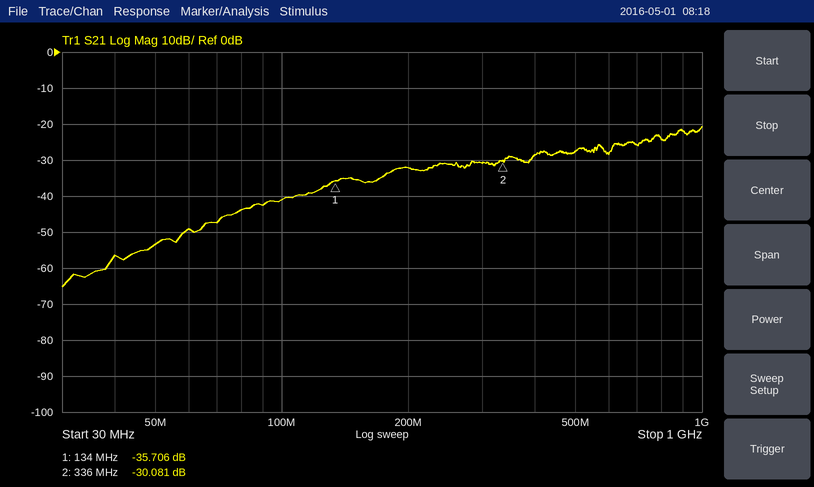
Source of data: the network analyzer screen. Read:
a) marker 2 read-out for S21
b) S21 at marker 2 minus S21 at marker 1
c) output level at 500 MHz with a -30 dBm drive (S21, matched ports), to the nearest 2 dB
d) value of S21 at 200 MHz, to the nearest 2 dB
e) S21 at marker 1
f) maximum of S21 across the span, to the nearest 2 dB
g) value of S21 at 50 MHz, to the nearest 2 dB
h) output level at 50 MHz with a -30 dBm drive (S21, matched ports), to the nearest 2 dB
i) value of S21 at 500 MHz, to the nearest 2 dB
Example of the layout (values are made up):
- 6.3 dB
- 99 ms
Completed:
- -30.081 dB
- 5.625 dB
- -58 dBm
- -32 dB
- -35.706 dB
- -20 dB
- -54 dB
- -84 dBm
- -28 dB
